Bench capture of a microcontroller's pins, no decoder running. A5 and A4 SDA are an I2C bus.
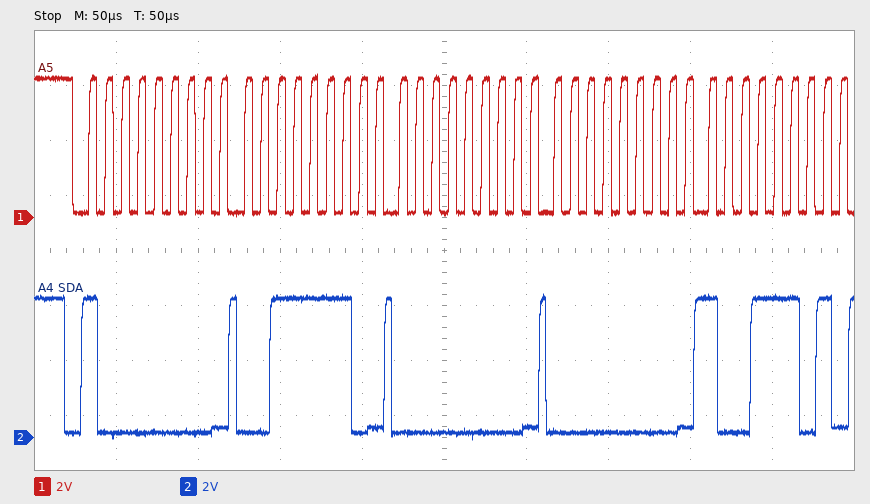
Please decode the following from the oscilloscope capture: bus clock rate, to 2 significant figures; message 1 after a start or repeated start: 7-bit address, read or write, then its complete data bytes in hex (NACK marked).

100 kHz
0x40 write: 3E 00 00 9D
